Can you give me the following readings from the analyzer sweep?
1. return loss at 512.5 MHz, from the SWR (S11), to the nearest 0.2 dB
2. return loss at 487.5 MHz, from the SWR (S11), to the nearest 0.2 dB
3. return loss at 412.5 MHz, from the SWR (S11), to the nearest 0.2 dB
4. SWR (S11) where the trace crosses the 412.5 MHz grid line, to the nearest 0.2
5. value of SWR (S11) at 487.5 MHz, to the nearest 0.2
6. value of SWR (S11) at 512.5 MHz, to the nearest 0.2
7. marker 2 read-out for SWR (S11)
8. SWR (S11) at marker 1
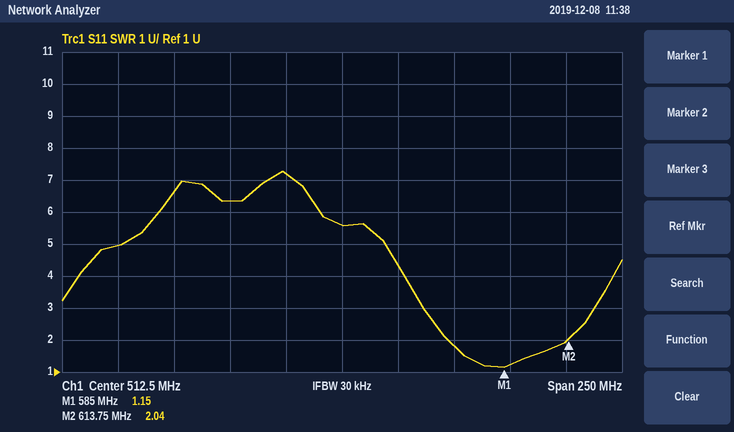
3.2 dB
2.4 dB
3.6 dB
5.0
7.2
5.6
2.04
1.15
